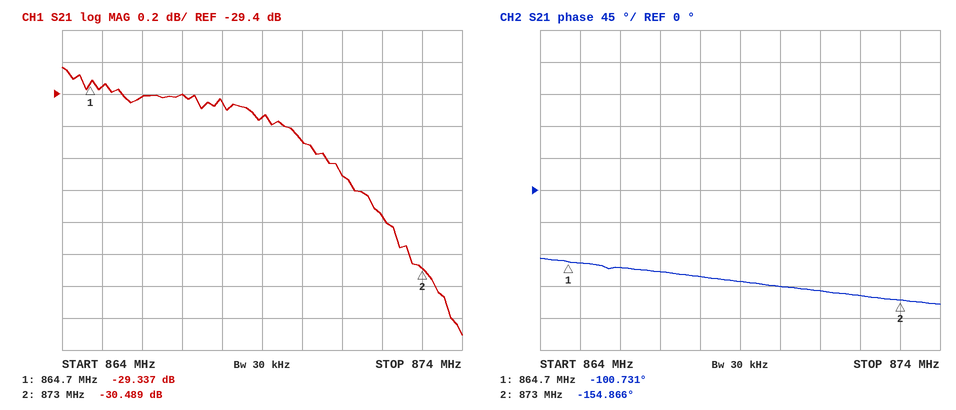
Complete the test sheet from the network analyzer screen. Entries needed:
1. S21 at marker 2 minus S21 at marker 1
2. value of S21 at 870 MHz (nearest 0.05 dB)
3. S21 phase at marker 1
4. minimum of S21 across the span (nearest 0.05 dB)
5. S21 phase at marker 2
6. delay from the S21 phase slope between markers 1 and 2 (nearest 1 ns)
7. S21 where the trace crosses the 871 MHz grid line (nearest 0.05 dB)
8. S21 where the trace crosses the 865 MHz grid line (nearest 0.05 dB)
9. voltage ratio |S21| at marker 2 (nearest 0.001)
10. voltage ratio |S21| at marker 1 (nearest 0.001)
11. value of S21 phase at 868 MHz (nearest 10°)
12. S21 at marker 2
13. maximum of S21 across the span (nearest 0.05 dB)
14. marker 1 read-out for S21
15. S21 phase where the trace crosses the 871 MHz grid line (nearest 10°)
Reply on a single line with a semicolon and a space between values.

-1.152 dB; -29.70 dB; -100.731°; -30.90 dB; -154.866°; 18 ns; -29.90 dB; -29.35 dB; 0.030; 0.034; -120°; -30.489 dB; -29.25 dB; -29.337 dB; -140°
